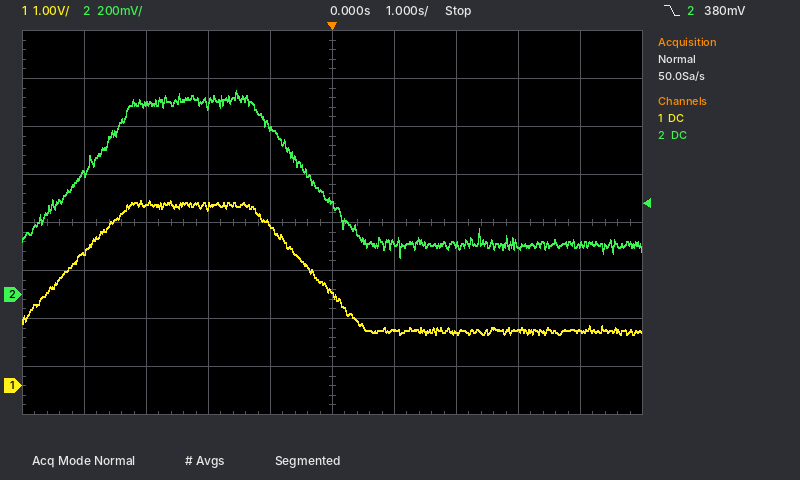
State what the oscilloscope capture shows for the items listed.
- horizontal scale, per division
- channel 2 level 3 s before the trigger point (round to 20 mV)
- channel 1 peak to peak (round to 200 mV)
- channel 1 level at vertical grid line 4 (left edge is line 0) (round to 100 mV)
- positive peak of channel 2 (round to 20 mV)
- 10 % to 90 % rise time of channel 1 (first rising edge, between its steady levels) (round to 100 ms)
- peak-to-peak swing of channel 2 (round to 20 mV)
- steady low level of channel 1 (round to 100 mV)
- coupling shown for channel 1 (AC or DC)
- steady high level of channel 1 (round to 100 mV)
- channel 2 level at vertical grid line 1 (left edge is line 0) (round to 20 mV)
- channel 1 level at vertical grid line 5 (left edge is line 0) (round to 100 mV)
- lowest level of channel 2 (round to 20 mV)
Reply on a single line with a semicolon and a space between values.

1 s; 800 mV; 2.8 V; 3.4 V; 860 mV; 1.5 s; 700 mV; 1.1 V; DC; 3.8 V; 500 mV; 1.9 V; 160 mV
